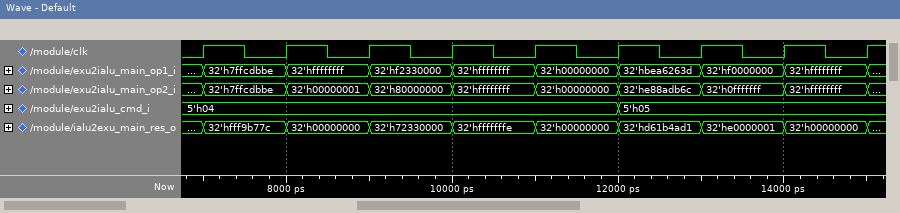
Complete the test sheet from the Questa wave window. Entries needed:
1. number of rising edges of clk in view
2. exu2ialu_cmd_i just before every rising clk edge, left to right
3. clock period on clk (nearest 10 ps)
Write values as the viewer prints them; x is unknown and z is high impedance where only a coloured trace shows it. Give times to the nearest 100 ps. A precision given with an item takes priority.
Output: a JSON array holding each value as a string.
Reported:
["9", "5'h04, 5'h04, 5'h04, 5'h04, 5'h04, 5'h04, 5'h05, 5'h05, 5'h05", "1000 ps"]
